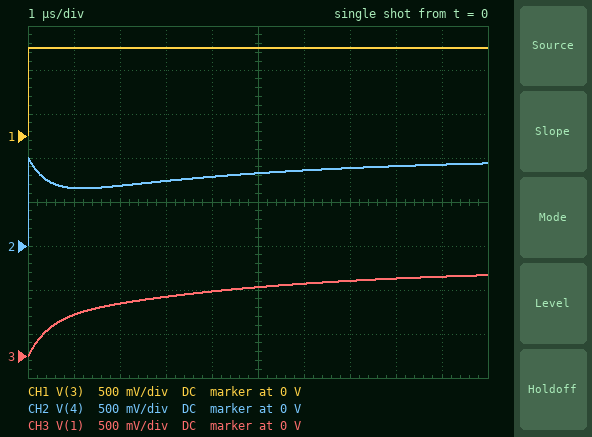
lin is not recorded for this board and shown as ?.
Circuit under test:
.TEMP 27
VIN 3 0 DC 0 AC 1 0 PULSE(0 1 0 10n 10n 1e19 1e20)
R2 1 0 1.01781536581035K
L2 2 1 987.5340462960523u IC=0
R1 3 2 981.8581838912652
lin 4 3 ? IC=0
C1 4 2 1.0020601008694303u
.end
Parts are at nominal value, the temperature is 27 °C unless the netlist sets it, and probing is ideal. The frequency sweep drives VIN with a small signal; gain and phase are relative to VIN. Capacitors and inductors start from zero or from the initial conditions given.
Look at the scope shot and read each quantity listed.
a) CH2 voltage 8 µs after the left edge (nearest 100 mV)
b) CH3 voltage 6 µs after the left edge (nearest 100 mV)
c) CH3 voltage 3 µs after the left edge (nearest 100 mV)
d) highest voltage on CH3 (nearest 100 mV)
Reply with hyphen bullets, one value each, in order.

- 900 mV
- 800 mV
- 700 mV
- 900 mV
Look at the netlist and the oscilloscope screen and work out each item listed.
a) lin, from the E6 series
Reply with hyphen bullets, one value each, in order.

- 2.2 mH
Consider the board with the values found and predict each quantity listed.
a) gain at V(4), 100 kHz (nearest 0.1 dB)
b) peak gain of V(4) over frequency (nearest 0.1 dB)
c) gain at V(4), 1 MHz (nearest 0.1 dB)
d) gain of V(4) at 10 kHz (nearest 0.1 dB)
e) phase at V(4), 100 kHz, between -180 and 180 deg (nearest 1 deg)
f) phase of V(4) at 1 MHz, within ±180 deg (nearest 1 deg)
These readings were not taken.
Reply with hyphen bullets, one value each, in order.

- -4.5 dB
- 0 dB
- -0.4 dB
- -0.3 dB
- -2 deg
- 8 deg
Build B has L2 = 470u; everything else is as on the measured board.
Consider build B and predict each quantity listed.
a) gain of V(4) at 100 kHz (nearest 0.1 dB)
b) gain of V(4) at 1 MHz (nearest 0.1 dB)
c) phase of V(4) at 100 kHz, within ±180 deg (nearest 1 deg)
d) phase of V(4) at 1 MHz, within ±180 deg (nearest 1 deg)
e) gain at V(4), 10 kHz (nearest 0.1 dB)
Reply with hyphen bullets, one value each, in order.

- -4.8 dB
- -1.3 dB
- -8 deg
- 14 deg
- -0.2 dB
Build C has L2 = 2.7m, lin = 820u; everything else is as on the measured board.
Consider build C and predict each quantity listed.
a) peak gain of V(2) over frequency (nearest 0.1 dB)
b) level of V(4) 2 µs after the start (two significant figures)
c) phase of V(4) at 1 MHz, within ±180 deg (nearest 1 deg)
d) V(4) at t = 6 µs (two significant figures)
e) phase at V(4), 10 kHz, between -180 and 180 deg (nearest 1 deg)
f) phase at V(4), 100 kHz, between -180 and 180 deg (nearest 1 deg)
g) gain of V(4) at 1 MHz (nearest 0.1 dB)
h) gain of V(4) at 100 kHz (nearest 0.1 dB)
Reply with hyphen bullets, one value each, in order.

- 0 dB
- 860 mV
- 3 deg
- 950 mV
- -3 deg
- -1 deg
- -0.1 dB
- -1.8 dB
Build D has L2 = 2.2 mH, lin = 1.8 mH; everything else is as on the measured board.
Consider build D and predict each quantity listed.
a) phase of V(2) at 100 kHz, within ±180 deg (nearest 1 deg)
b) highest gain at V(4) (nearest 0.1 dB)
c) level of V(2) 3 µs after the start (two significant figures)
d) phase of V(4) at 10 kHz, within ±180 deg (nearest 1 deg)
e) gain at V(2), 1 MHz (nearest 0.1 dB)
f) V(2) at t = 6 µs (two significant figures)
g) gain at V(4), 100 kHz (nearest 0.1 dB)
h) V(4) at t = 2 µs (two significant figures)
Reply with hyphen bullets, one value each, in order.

- 4 deg
- 0 dB
- 780 mV
- -6 deg
- -0.1 dB
- 870 mV
- -3.1 dB
- 750 mV
